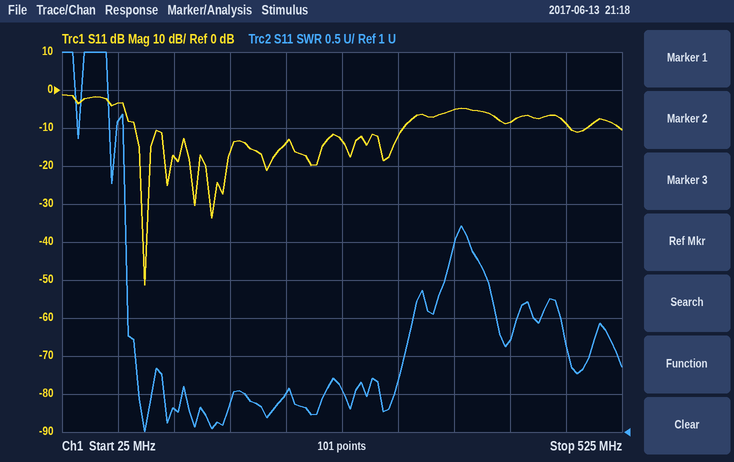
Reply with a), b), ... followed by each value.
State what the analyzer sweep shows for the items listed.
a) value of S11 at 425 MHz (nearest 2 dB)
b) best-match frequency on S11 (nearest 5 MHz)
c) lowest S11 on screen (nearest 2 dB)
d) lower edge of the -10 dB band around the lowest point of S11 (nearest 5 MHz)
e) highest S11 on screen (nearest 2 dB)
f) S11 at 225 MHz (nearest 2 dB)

a) -8 dB
b) 100 MHz
c) -52 dB
d) 90 MHz
e) -2 dB
f) -14 dB
